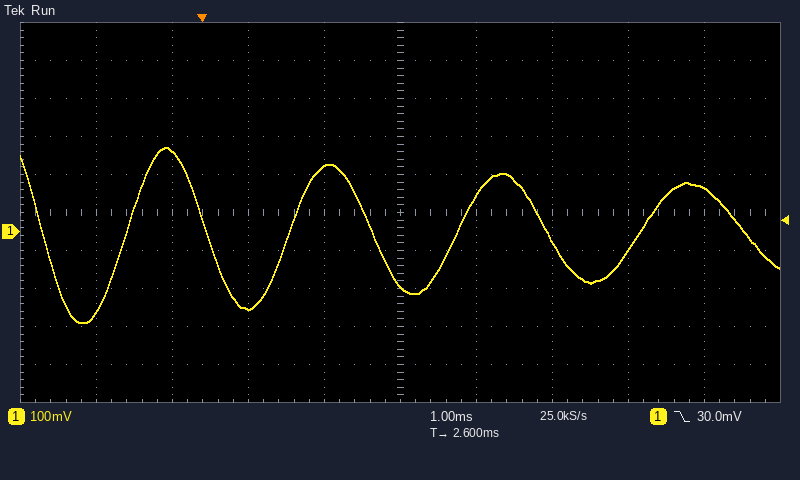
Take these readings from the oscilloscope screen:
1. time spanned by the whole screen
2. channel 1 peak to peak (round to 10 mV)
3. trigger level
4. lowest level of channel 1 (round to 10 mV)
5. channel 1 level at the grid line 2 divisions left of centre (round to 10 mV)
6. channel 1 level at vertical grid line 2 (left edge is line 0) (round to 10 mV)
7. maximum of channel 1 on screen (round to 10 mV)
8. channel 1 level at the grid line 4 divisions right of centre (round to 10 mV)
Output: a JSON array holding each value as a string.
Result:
["10 ms", "460 mV", "30.0 mV", "-240 mV", "-200 mV", "210 mV", "220 mV", "110 mV"]
